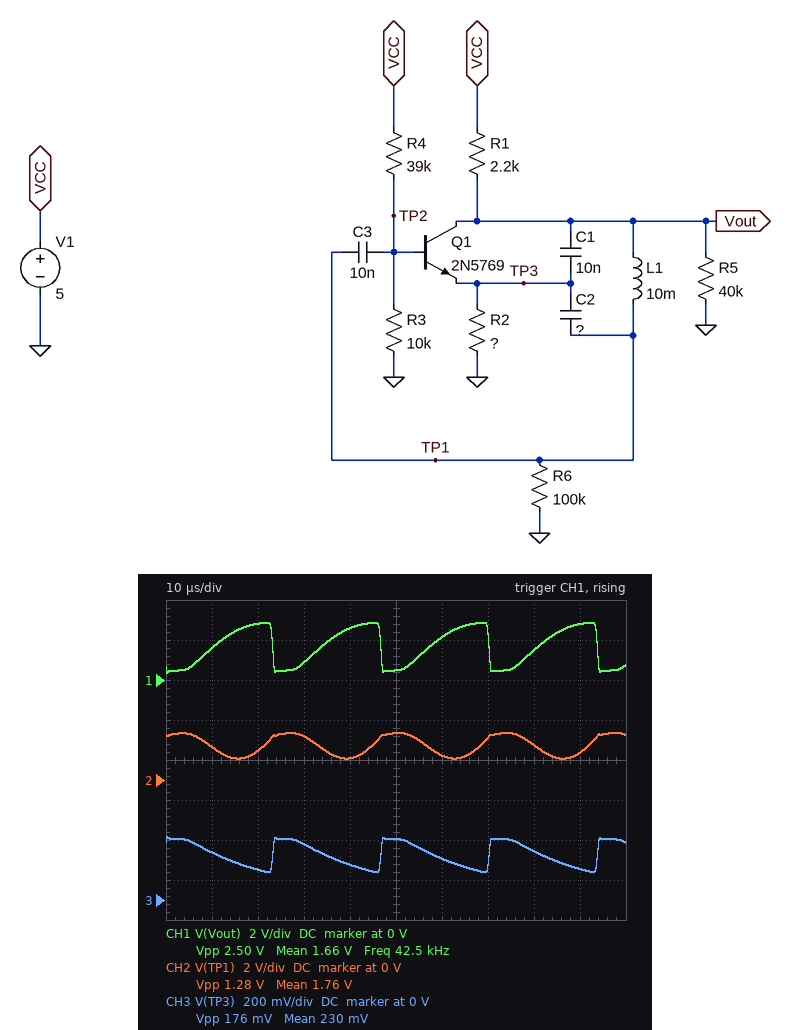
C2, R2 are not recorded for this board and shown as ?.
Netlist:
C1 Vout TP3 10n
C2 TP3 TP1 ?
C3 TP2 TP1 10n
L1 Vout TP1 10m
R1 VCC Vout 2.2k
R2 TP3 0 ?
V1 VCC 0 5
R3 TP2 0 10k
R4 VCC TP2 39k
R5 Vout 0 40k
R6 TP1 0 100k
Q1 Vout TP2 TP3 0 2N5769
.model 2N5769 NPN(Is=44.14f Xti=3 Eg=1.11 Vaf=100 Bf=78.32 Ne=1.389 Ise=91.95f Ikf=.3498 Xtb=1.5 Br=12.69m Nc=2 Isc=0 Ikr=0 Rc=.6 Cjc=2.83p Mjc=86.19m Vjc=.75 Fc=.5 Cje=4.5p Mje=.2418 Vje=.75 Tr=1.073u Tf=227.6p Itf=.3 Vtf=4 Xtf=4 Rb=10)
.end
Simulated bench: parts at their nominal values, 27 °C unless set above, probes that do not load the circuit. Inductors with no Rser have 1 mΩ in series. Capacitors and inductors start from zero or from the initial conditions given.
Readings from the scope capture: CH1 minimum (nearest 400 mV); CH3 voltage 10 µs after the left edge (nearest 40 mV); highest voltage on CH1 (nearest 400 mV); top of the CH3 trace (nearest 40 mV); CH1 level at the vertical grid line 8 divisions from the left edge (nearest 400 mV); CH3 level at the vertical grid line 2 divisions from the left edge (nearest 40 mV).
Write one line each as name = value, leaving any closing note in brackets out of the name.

CH1 minimum = 400 mV
CH3 voltage 10 µs after the left edge = 240 mV
highest voltage on CH1 = 2.8 V
top of the CH3 trace = 320 mV
CH1 level at the vertical grid line 8 divisions from the left edge = 1.6 V
CH3 level at the vertical grid line 2 divisions from the left edge = 160 mV
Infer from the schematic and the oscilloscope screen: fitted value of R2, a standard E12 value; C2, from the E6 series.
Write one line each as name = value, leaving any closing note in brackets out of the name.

fitted value of R2, a standard E12 value = 150 Ω
C2, from the E6 series = 3.3 nF
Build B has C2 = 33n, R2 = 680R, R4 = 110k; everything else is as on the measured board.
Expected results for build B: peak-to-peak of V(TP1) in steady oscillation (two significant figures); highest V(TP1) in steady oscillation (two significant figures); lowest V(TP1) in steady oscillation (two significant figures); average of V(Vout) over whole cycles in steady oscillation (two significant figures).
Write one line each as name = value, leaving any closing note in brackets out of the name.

peak-to-peak of V(TP1) in steady oscillation = 2.4 V
highest V(TP1) in steady oscillation = 5.0 V
lowest V(TP1) in steady oscillation = 2.6 V
average of V(Vout) over whole cycles in steady oscillation = 3.7 V
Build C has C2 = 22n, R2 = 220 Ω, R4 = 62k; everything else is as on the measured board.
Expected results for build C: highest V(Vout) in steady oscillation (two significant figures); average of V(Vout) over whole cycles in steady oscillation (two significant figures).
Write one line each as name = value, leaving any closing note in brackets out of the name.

highest V(Vout) in steady oscillation = 4.8 V
average of V(Vout) over whole cycles in steady oscillation = 3.1 V
